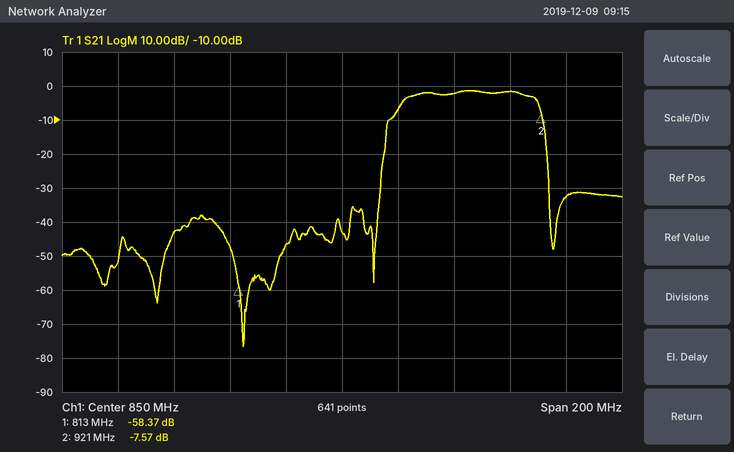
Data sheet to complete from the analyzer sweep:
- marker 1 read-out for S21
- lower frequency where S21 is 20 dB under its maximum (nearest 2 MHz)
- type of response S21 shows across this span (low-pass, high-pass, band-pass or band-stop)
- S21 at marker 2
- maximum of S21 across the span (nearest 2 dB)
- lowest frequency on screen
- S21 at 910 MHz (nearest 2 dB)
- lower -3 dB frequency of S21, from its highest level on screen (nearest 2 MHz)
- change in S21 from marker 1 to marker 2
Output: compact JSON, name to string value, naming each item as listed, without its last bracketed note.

{"marker 1 read-out for S21": "-58.37 dB", "lower frequency where S21 is 20 dB under its maximum": "864 MHz", "type of response S21 shows across this span": "band-pass", "S21 at marker 2": "-7.57 dB", "maximum of S21 across the span": "-2 dB", "lowest frequency on screen": "750 MHz", "S21 at 910 MHz": "-2 dB", "lower -3 dB frequency of S21, from its highest level on screen": "872 MHz", "change in S21 from marker 1 to marker 2": "50.80 dB"}
